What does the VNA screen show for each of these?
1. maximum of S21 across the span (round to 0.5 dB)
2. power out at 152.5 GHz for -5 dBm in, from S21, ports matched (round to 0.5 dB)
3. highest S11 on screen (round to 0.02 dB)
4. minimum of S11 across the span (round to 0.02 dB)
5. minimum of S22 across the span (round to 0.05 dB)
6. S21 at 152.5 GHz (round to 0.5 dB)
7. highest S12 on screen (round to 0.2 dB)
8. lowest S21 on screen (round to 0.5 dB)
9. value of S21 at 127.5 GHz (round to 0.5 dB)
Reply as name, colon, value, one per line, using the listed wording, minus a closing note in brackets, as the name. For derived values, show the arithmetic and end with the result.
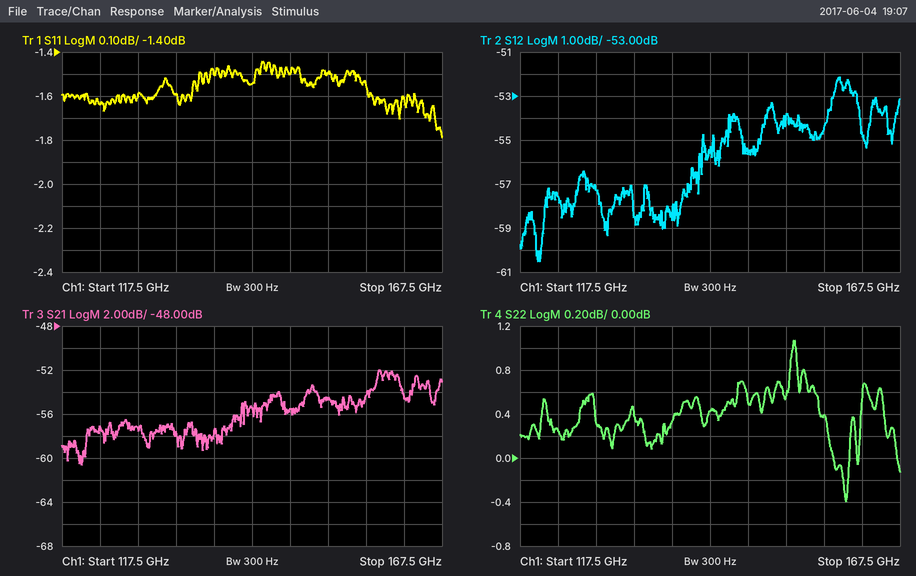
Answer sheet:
maximum of S21 across the span: -52.0 dB
power out at 152.5 GHz for -5 dBm in, from S21, ports matched: -5 dBm + (-54.5 dB) = -59.5 dBm
highest S11 on screen: -1.44 dB
minimum of S11 across the span: -1.78 dB
minimum of S22 across the span: -0.40 dB
S21 at 152.5 GHz: -54.5 dB
highest S12 on screen: -52.2 dB
lowest S21 on screen: -60.5 dB
value of S21 at 127.5 GHz: -57.5 dB
